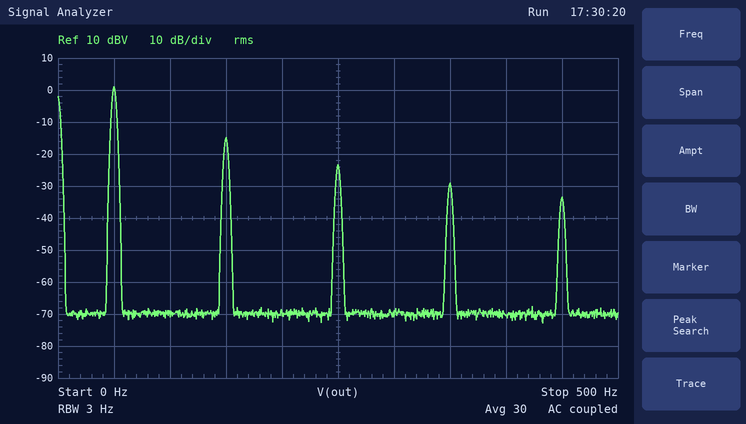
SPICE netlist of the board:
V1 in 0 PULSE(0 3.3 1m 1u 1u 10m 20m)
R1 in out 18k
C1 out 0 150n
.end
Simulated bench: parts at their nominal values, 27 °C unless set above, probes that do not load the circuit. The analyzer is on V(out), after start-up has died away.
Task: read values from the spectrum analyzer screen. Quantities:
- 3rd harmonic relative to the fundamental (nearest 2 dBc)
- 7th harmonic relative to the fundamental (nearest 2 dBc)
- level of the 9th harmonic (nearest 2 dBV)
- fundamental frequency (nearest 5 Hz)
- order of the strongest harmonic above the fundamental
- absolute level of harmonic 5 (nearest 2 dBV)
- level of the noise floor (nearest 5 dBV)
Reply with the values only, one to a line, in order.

-16 dBc
-30 dBc
-34 dBV
50 Hz
3
-24 dBV
-70 dBV
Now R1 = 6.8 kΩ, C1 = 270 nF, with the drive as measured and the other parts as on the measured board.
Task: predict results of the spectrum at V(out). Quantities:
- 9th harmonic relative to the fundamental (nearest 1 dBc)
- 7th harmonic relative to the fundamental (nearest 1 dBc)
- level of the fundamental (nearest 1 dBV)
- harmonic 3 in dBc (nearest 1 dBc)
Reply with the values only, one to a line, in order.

-32 dBc
-28 dBc
2 dBV
-14 dBc
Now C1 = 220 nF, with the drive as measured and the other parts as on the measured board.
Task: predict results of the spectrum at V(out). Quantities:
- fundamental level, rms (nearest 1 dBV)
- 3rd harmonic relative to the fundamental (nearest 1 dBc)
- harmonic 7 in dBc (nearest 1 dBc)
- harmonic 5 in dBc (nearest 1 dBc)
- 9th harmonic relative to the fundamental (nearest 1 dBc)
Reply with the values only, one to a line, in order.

-1 dBV
-17 dBc
-32 dBc
-26 dBc
-36 dBc
